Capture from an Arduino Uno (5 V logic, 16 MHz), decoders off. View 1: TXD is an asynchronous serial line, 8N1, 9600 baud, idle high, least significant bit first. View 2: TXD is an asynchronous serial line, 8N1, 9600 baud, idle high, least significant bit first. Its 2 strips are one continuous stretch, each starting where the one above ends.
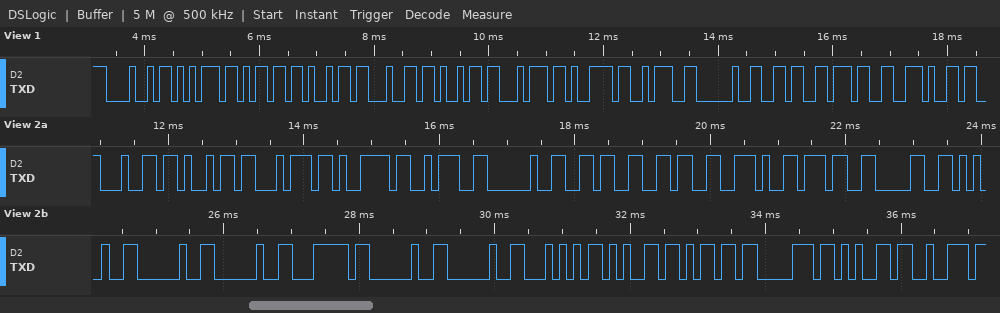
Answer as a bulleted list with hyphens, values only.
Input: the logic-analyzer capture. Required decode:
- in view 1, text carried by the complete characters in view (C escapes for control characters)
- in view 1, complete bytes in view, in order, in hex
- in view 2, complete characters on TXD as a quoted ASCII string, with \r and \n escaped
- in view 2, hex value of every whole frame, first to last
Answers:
- "Humidity: 67."
- 48 75 6D 69 64 69 74 79 3A 20 36 37 2E
- "dity: 66.70%  |  Temper"
- 0x64 0x69 0x74 0x79 0x3A 0x20 0x36 0x36 0x2E 0x37 0x30 0x25 0x20 0x20 0x7C 0x20 0x20 0x54 0x65 0x6D 0x70 0x65 0x72
